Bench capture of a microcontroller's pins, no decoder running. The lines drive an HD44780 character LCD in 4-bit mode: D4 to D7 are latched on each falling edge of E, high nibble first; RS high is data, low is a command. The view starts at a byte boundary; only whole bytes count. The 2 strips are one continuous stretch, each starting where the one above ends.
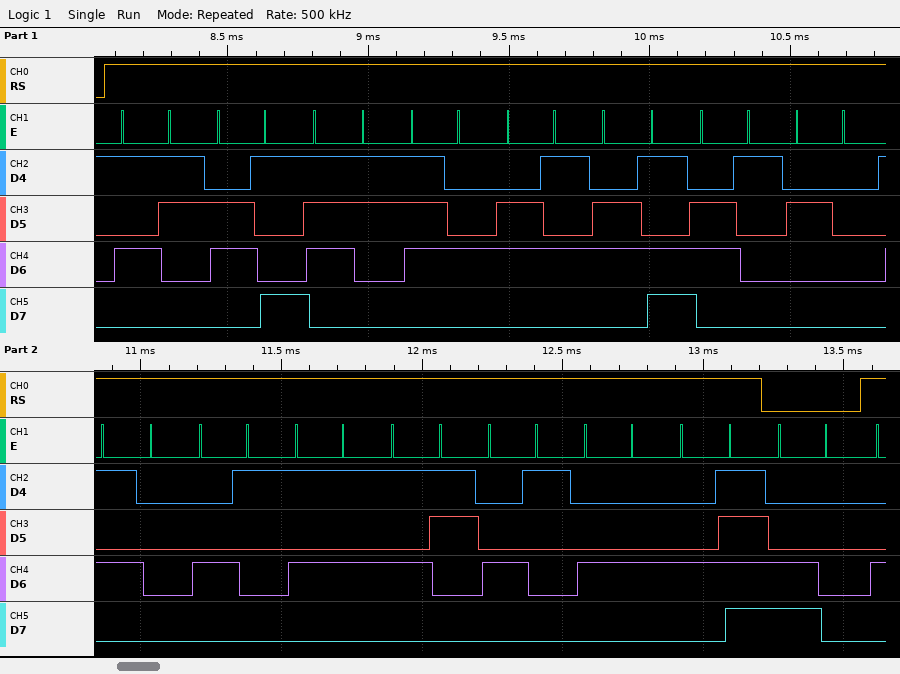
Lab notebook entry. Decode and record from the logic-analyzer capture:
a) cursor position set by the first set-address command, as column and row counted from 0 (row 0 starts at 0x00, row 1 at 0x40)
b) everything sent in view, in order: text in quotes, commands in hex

column 0, row 1
"Sistema PAUSADO" 0xC0
